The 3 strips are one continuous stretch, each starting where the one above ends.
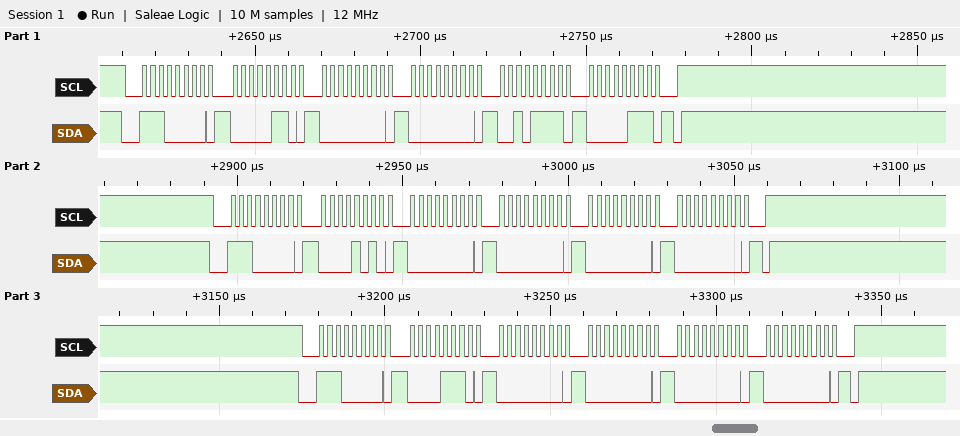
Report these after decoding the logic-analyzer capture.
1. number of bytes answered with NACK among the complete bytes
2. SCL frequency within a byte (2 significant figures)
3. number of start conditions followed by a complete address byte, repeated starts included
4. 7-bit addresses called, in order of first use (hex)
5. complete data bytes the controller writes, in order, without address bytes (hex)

0
400 kHz
3
0x70
06 00 00 2F 07 0A 00 00 00 00 0E 00 00 00 00
